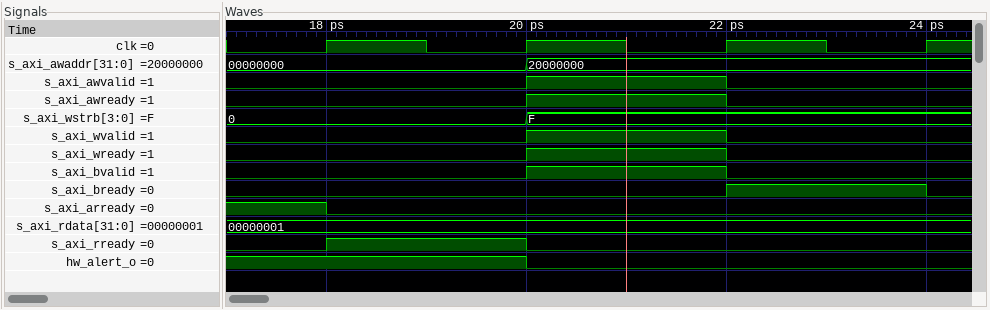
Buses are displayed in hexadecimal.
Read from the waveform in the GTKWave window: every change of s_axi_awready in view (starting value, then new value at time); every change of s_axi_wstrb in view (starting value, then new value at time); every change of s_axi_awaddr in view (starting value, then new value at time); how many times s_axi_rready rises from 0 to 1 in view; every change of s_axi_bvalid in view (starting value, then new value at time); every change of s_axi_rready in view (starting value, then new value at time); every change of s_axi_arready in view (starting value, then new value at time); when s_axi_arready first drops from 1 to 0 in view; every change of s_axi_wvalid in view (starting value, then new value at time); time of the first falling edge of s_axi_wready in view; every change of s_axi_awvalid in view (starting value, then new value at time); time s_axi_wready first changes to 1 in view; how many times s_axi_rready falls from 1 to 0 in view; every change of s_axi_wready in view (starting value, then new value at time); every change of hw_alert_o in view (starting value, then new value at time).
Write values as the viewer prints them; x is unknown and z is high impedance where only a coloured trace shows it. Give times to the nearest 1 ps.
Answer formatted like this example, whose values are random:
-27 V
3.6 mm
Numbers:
0, 1 at 20 ps, 0 at 22 ps
0, F at 20 ps
00000000, 20000000 at 20 ps
1
0, 1 at 20 ps, 0 at 22 ps
0, 1 at 18 ps, 0 at 20 ps
1, 0 at 18 ps
18 ps
0, 1 at 20 ps, 0 at 22 ps
22 ps
0, 1 at 20 ps, 0 at 22 ps
20 ps
1
0, 1 at 20 ps, 0 at 22 ps
1, 0 at 20 ps
